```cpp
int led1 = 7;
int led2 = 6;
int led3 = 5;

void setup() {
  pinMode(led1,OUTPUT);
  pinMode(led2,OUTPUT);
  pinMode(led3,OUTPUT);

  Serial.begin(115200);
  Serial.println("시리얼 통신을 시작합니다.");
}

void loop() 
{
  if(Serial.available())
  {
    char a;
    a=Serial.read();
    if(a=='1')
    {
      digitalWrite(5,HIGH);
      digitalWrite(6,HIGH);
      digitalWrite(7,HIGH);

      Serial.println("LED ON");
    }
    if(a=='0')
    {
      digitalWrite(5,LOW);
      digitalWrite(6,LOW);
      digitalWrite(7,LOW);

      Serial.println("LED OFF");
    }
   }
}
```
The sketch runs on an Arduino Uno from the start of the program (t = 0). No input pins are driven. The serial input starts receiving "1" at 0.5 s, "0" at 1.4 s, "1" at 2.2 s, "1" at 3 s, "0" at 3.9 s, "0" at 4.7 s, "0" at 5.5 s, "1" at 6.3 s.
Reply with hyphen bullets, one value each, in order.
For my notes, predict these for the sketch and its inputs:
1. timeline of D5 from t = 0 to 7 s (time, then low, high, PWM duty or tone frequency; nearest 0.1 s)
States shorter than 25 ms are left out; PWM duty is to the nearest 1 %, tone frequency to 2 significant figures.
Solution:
- 0 s low; 0.5 s high; 1.4 s low; 2.2 s high; 3.9 s low; 6.3 s high
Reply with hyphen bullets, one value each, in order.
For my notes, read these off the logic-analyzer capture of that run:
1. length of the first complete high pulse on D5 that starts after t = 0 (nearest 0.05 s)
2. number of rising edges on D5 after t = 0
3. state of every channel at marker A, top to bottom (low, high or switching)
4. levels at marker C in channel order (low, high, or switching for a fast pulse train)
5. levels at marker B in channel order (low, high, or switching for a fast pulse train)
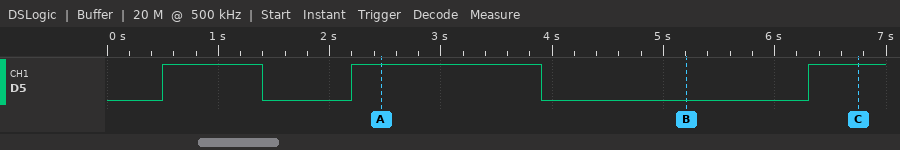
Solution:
- 0.90 s
- 3
- D5 high
- D5 high
- D5 low
